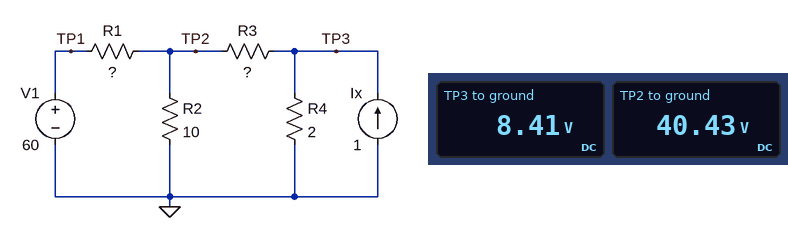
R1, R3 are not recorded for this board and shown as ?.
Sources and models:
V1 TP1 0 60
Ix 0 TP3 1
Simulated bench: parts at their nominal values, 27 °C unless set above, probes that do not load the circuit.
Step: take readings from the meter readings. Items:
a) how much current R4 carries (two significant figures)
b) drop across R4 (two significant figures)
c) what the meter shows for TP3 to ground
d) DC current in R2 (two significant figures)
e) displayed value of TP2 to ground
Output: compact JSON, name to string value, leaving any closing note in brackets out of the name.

{"how much current R4 carries": "4.2 A", "drop across R4": "8.4 V", "what the meter shows for TP3 to ground": "8.41 V", "DC current in R2": "4.0 A", "displayed value of TP2 to ground": "40.43 V"}
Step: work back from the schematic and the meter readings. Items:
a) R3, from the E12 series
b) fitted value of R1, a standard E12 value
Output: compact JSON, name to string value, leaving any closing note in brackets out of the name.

{"R3, from the E12 series": "10 Ω", "fitted value of R1, a standard E12 value": "2.7 Ω"}
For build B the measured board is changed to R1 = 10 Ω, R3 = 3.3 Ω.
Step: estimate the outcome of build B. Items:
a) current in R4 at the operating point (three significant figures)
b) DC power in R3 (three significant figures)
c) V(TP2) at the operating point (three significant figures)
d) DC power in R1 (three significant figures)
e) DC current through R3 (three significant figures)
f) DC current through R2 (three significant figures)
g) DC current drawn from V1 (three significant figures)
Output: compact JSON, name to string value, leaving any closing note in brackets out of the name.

{"current in R4 at the operating point": "3.72 A", "DC power in R3": "24.4 W", "V(TP2) at the operating point": "16.4 V", "DC power in R1": "190 W", "DC current through R3": "2.72 A", "DC current through R2": "1.64 A", "DC current drawn from V1": "4.36 A"}
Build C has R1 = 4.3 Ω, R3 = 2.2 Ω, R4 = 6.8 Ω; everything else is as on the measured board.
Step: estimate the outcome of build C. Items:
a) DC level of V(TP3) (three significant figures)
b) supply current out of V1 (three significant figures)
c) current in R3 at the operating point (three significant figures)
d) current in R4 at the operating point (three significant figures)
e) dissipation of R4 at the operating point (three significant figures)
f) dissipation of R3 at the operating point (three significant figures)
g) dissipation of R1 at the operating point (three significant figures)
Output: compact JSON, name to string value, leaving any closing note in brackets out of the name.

{"DC level of V(TP3)": "26.7 V", "supply current out of V1": "6.24 A", "current in R3 at the operating point": "2.93 A", "current in R4 at the operating point": "3.93 A", "dissipation of R4 at the operating point": "105 W", "dissipation of R3 at the operating point": "18.9 W", "dissipation of R1 at the operating point": "168 W"}
